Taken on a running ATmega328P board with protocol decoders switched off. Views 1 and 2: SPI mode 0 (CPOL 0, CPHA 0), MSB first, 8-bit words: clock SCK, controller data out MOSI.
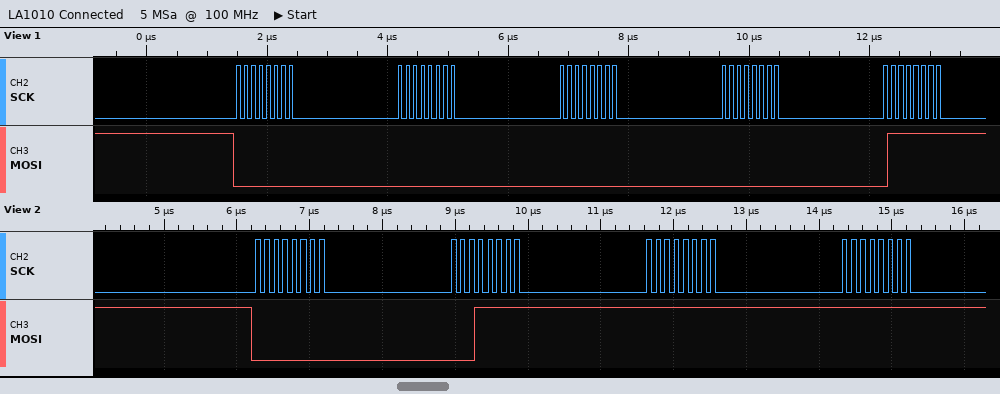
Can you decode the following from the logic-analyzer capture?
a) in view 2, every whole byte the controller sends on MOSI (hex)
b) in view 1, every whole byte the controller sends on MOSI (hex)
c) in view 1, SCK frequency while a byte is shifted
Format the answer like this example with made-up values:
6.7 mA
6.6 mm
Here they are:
0x00 0x1F 0xFF 0xFF
00 00 00 00 7F
8 MHz
